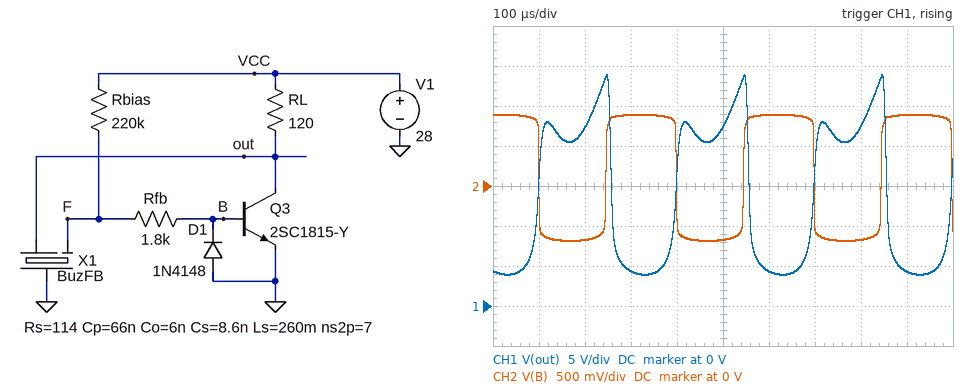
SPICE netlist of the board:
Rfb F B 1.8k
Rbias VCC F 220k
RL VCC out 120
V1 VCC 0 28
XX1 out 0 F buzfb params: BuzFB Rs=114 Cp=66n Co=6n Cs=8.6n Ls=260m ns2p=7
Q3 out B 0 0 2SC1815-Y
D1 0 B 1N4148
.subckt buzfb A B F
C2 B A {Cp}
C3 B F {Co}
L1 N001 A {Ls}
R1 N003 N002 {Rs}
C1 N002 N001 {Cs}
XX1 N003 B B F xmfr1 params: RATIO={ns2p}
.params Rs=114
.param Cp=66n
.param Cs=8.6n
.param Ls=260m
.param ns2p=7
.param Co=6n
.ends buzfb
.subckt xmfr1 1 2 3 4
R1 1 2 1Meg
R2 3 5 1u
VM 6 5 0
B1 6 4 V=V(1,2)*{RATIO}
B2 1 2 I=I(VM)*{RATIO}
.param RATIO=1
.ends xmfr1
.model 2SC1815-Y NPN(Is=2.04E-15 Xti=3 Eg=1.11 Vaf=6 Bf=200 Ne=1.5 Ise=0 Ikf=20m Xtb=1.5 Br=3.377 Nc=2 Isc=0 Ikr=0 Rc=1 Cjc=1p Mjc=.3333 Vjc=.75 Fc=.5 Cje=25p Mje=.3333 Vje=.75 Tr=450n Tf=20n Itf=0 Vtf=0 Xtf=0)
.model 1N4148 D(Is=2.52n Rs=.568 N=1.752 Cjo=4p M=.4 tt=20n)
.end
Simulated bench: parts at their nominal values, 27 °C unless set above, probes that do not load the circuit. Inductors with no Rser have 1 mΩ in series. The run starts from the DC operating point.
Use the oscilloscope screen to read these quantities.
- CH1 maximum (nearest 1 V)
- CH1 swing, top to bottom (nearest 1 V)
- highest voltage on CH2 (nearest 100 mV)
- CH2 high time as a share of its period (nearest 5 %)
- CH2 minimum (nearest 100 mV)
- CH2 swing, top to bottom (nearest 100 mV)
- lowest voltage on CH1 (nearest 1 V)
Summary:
29 V
25 V
900 mV
50 %
-700 mV
1.6 V
4 V
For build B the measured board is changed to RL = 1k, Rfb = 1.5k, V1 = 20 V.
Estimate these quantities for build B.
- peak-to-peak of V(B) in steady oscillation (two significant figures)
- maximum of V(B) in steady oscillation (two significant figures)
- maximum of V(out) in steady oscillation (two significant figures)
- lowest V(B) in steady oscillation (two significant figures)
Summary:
1.5 V
840 mV
13 V
-620 mV
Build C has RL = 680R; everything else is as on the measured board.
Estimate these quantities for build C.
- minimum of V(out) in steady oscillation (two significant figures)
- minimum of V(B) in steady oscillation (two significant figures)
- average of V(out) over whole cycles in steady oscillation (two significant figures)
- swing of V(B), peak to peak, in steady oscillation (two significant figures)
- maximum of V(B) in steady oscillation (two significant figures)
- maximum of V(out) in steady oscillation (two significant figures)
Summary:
160 mV
-650 mV
6.2 V
1.5 V
850 mV
21 V
